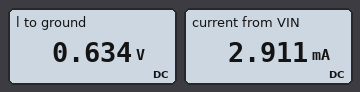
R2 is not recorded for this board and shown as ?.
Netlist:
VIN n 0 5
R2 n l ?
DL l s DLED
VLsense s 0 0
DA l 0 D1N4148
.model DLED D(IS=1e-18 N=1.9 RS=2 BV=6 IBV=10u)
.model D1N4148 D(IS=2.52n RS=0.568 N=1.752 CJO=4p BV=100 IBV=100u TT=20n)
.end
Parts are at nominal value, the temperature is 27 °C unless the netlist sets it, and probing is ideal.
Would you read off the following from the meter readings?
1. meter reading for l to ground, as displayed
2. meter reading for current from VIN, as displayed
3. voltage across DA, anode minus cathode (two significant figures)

0.634 V
2.911 mA
630 mV
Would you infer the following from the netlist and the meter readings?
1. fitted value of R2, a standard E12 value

1.5 kΩ
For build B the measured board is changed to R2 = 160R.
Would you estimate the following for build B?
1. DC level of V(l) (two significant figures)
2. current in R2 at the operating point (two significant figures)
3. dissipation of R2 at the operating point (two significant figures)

750 mV
27 mA
110 mW
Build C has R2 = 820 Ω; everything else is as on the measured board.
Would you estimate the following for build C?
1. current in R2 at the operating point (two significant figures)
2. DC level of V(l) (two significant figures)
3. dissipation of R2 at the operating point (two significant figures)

5.3 mA
660 mV
23 mW
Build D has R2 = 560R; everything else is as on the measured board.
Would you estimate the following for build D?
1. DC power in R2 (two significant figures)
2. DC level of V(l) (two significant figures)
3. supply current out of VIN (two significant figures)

33 mW
680 mV
7.7 mA
